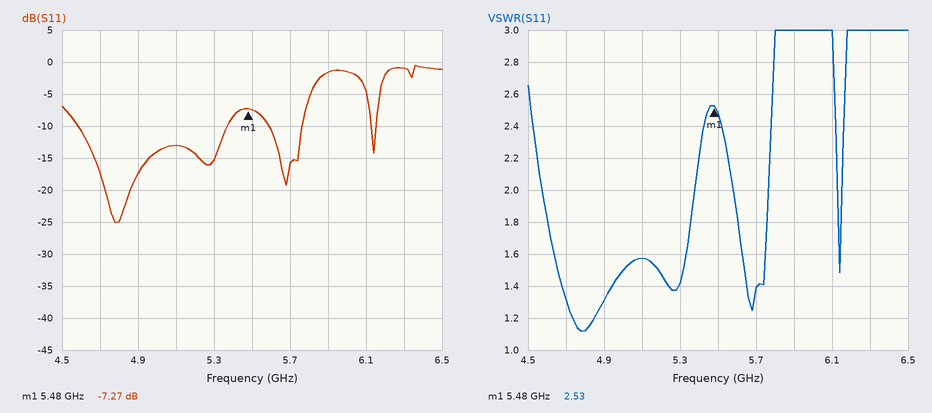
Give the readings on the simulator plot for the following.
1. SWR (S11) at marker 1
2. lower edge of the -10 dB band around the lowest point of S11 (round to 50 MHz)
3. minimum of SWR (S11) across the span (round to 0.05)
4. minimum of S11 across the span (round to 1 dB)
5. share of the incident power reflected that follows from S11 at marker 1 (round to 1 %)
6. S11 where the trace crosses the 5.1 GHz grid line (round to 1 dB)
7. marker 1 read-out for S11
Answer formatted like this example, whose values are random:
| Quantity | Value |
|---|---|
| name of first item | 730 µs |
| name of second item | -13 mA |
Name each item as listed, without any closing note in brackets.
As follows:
| Quantity | Value |
|---|---|
| SWR (S11) at marker 1 | 2.53 |
| lower edge of the -10 dB band around the lowest point of S11 | 4.60 GHz |
| minimum of SWR (S11) across the span | 1.10 |
| minimum of S11 across the span | -25 dB |
| share of the incident power reflected that follows from S11 at marker 1 | 19 % |
| S11 where the trace crosses the 5.1 GHz grid line | -13 dB |
| marker 1 read-out for S11 | -7.27 dB |
